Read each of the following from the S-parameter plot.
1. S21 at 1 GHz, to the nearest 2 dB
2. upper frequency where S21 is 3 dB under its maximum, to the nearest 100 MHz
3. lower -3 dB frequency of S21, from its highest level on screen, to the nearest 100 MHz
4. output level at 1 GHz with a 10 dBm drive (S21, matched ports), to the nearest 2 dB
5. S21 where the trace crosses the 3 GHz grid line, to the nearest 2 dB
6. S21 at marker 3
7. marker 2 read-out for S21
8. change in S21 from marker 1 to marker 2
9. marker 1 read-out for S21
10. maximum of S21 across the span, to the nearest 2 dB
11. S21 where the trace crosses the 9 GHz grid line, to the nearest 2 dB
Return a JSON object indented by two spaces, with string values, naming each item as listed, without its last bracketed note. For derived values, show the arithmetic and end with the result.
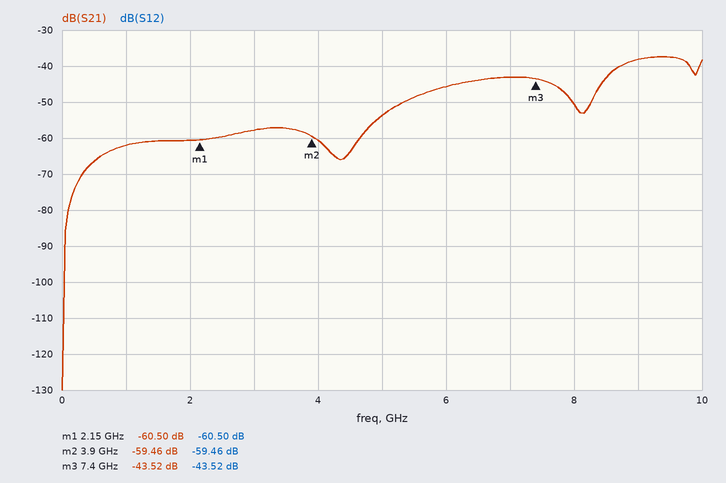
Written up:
{
  "S21 at 1 GHz, to the nearest 2 dB": "-62 dB",
  "upper frequency where S21 is 3 dB under its maximum, to the nearest 100 MHz": "9.8 GHz",
  "lower -3 dB frequency of S21, from its highest level on screen, to the nearest 100 MHz": "8.7 GHz",
  "output level at 1 GHz with a 10 dBm drive (S21, matched ports), to the nearest 2 dB": "10 dBm + (-62 dB) = -52 dBm",
  "S21 where the trace crosses the 3 GHz grid line, to the nearest 2 dB": "-58 dB",
  "S21 at marker 3": "-43.52 dB",
  "marker 2 read-out for S21": "-59.46 dB",
  "change in S21 from marker 1 to marker 2": "-59.46 − (-60.5) = 1.04 dB",
  "marker 1 read-out for S21": "-60.50 dB",
  "maximum of S21 across the span, to the nearest 2 dB": "-38 dB",
  "S21 where the trace crosses the 9 GHz grid line, to the nearest 2 dB": "-38 dB"
}
